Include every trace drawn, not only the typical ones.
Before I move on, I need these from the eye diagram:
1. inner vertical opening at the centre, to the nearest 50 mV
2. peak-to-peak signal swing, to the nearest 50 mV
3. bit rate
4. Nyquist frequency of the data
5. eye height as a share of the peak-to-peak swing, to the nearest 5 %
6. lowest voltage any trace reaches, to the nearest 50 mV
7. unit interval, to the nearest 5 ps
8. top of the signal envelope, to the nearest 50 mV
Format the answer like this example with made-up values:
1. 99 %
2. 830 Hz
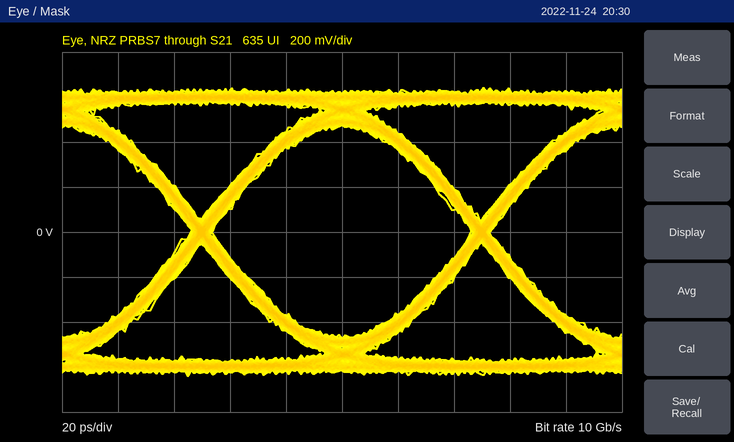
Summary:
1. 950 mV
2. 1.30 V
3. 10 Gb/s
4. 5 GHz
5. 75 %
6. -650 mV
7. 100 ps
8. 650 mV
